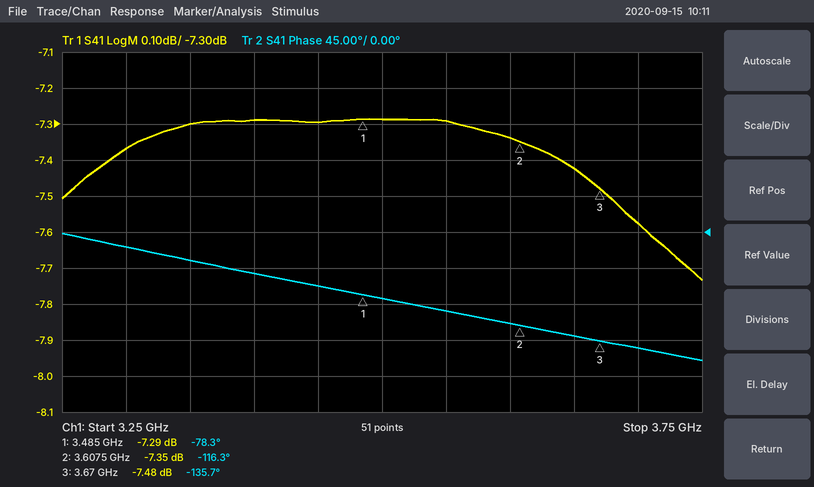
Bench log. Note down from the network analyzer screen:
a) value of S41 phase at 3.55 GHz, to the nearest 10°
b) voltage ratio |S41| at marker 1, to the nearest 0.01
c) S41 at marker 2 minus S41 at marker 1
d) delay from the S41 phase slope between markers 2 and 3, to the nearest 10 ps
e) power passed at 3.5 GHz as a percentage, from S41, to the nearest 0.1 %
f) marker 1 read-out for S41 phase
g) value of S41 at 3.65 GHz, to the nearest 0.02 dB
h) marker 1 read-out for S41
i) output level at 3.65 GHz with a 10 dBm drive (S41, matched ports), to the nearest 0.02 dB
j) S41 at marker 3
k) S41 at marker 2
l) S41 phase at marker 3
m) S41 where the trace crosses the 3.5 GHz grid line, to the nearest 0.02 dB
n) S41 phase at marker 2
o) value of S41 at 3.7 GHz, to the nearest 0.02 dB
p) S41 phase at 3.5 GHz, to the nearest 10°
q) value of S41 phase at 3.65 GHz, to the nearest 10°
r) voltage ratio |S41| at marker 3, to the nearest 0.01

-100°
0.43
-0.06 dB
860 ps
18.7 %
-78.3°
-7.42 dB
-7.29 dB
2.58 dBm
-7.48 dB
-7.35 dB
-135.7°
-7.28 dB
-116.3°
-7.58 dB
-80°
-130°
0.42
